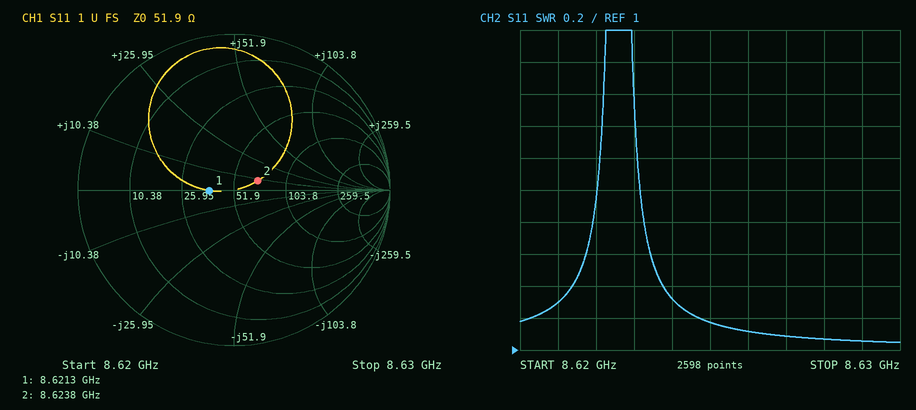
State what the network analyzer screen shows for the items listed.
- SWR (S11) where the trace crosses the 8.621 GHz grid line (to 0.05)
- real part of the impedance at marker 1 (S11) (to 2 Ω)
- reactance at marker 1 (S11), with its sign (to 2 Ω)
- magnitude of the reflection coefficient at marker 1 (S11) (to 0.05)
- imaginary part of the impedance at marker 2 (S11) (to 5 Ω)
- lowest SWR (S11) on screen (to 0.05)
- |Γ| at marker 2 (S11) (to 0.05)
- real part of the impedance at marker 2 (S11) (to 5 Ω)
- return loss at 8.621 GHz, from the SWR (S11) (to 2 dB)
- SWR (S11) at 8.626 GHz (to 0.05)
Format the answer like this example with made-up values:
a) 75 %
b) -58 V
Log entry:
a) 1.30
b) 38 Ω
c) 0 Ω
d) 0.15
e) +10 Ω
f) 1.05
g) 0.15
h) 70 Ω
i) 18 dB
j) 1.10
